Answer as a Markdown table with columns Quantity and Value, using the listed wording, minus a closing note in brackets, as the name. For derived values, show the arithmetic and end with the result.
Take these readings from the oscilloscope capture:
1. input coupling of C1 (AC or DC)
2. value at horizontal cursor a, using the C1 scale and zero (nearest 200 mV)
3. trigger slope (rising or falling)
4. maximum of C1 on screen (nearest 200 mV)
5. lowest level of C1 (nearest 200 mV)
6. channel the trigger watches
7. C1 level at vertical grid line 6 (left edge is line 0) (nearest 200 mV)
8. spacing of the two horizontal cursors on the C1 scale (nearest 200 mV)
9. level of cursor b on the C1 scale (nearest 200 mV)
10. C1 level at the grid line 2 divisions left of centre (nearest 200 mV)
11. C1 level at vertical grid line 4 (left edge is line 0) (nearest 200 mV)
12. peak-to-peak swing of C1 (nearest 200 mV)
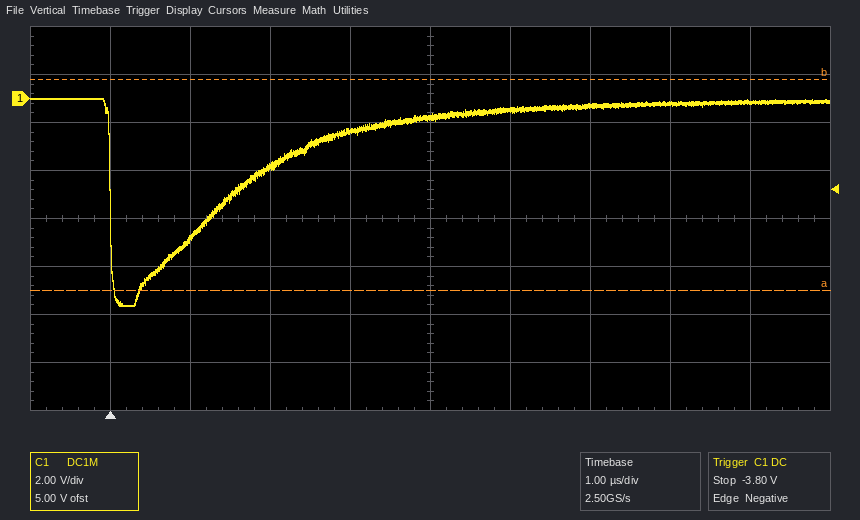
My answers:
| Quantity | Value |
|---|---|
| input coupling of C1 | DC |
| value at horizontal cursor a, using the C1 scale and zero | -8.0 V |
| trigger slope | falling |
| maximum of C1 on screen | 0.0 V |
| lowest level of C1 | -8.6 V |
| channel the trigger watches | C1 |
| C1 level at vertical grid line 6 (left edge is line 0) | -400 mV |
| spacing of the two horizontal cursors on the C1 scale | 8.8 V |
| level of cursor b on the C1 scale | 800 mV |
| C1 level at the grid line 2 divisions left of centre | -2.8 V |
| C1 level at vertical grid line 4 (left edge is line 0) | -1.4 V |
| peak-to-peak swing of C1 | 0.0 V − (-8.6 V) = 8.6 V |
